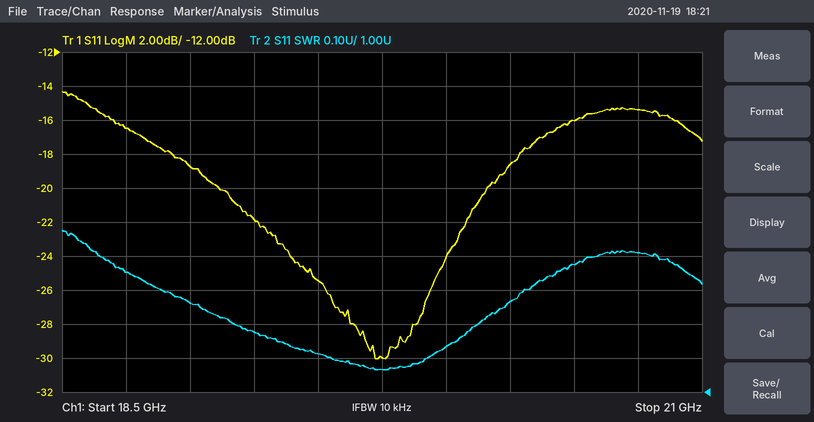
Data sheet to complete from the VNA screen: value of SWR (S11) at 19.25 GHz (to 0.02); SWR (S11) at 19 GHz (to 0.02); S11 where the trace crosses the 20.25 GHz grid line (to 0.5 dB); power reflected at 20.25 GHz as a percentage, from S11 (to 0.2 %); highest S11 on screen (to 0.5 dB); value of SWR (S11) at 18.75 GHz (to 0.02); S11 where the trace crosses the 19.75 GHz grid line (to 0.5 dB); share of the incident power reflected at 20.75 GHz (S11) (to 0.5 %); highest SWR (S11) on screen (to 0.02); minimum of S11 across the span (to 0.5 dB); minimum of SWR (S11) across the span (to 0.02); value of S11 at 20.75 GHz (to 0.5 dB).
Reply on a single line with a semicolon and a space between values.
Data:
1.18; 1.26; -18.5 dB; 1.4 %; -14.5 dB; 1.36; -30.0 dB; 3.0 %; 1.48; -30.0 dB; 1.06; -15.5 dB
